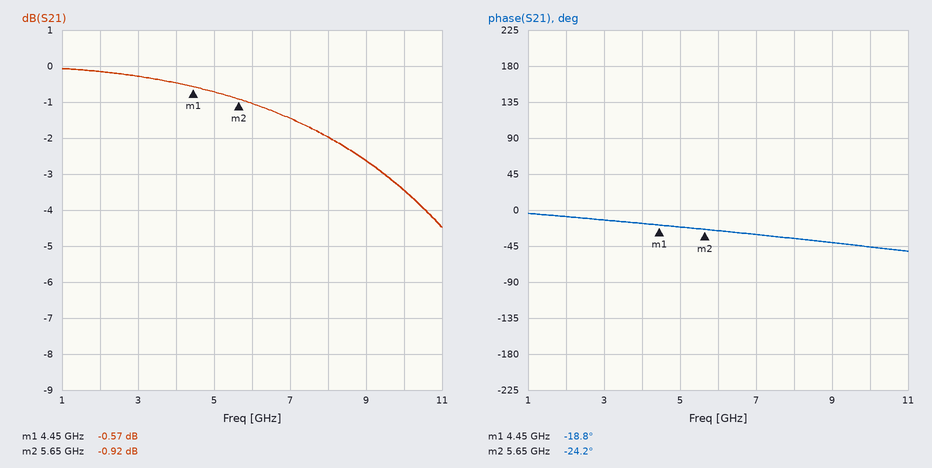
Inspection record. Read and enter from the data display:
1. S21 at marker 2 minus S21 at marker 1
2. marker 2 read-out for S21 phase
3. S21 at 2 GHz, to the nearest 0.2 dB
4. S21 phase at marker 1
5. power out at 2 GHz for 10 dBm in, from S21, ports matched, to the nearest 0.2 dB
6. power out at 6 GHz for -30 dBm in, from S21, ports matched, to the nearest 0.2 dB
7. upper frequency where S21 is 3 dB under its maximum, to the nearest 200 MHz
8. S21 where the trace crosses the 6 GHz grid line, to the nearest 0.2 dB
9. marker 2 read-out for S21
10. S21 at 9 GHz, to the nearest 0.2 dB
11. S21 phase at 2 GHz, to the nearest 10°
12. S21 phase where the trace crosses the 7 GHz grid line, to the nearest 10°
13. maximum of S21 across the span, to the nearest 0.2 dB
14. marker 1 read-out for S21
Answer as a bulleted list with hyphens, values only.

- -0.35 dB
- -24.2°
- -0.2 dB
- -18.8°
- 9.8 dBm
- -31.0 dBm
- 9.6 GHz
- -1.0 dB
- -0.92 dB
- -2.6 dB
- -10°
- -30°
- 0.0 dB
- -0.57 dB
